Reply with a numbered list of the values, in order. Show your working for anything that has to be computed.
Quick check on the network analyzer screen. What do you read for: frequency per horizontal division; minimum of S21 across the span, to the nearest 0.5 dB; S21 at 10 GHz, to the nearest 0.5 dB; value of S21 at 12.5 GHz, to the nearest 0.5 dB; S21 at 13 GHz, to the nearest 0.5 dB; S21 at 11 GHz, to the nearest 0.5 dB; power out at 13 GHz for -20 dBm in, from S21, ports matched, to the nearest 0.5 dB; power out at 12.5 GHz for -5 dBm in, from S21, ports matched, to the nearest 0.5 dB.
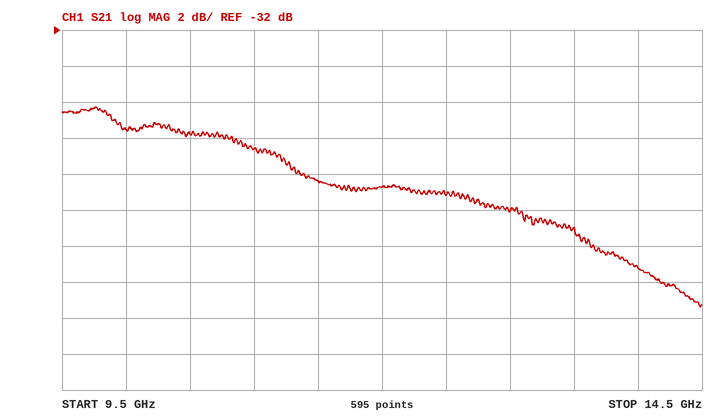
1. 500 MHz
2. -47.5 dB
3. -37.5 dB
4. -41.0 dB
5. -42.0 dB
6. -38.5 dB
7. -20 dBm + (-42.0 dB) = -62.0 dBm
8. -5 dBm + (-41.0 dB) = -46.0 dBm
